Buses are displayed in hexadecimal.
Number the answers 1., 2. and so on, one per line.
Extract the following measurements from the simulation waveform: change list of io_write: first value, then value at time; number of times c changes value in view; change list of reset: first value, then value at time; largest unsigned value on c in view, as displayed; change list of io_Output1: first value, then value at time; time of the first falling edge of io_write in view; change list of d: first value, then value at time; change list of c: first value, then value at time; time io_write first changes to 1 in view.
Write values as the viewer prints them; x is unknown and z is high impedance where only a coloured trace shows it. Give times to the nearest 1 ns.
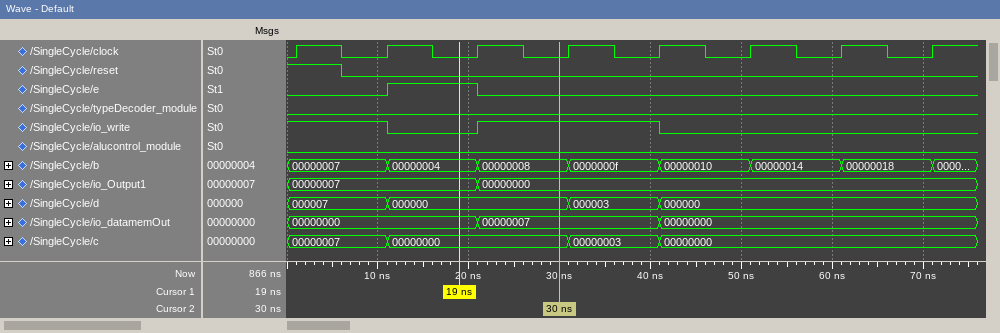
1. 1, 0 at 11 ns, 1 at 21 ns, 0 at 41 ns
2. 3
3. 1, 0 at 6 ns
4. 00000007
5. 00000007, 00000000 at 21 ns
6. 11 ns
7. 000007, 000000 at 11 ns, 000003 at 31 ns, 000000 at 41 ns
8. 00000007, 00000000 at 11 ns, 00000003 at 31 ns, 00000000 at 41 ns
9. 21 ns
